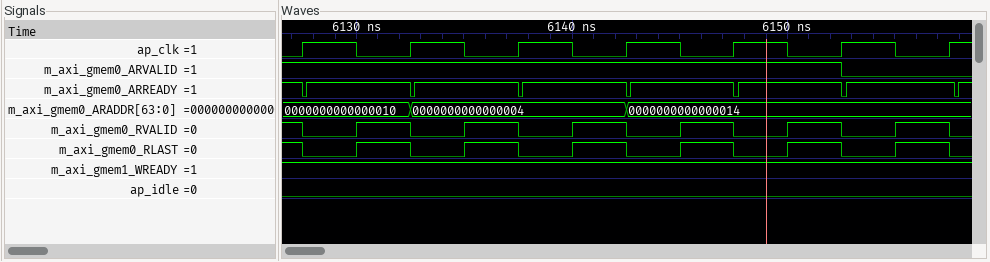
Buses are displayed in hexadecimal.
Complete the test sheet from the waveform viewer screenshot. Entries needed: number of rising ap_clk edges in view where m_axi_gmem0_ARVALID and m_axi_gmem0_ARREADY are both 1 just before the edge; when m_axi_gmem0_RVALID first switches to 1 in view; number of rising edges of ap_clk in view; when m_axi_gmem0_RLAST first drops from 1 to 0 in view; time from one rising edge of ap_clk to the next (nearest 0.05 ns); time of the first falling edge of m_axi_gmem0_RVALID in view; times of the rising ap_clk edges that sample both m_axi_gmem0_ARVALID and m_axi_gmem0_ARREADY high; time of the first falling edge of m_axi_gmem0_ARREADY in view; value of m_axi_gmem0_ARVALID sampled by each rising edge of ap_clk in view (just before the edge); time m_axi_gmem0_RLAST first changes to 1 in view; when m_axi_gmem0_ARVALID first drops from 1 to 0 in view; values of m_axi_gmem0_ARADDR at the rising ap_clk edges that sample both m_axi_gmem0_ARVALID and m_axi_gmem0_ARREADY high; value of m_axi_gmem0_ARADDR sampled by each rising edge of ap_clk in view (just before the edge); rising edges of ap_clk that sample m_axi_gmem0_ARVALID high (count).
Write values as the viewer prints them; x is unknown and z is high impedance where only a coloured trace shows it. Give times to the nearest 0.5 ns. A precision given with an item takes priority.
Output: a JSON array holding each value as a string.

["6", "6130 ns", "7", "6127.5 ns", "5 ns", "6127.5 ns", "6127.5 ns, 6132.5 ns, 6137.5 ns, 6142.5 ns, 6147.5 ns, 6152.5 ns", "6127.5 ns", "1 1 1 1 1 1 0", "6130 ns", "6152.5 ns", "0000000000000010, 0000000000000010, 0000000000000004, 0000000000000004, 0000000000000014, 0000000000000014", "0000000000000010, 0000000000000010, 0000000000000004, 0000000000000004, 0000000000000014, 0000000000000014, 0000000000000014", "6"]
